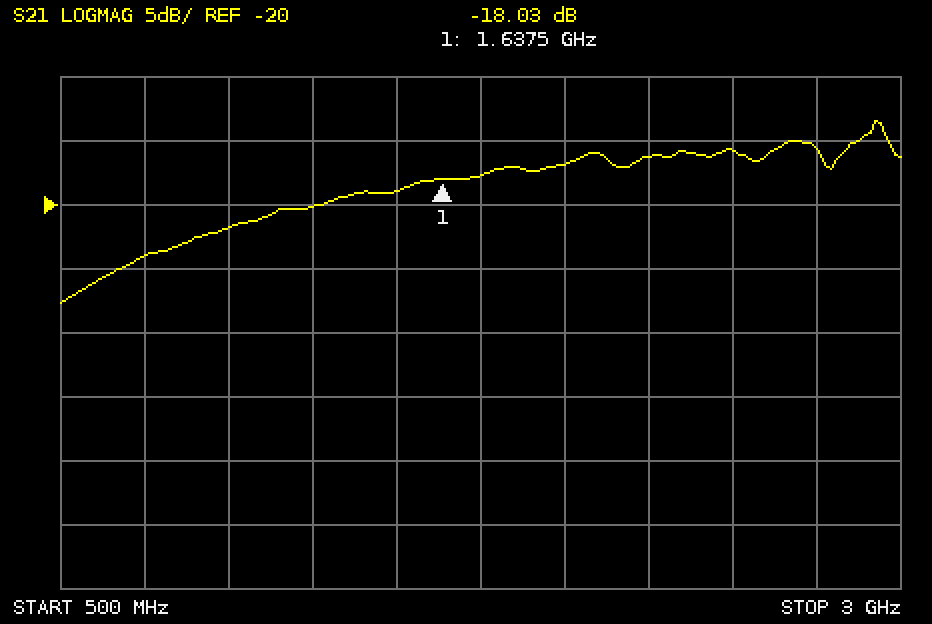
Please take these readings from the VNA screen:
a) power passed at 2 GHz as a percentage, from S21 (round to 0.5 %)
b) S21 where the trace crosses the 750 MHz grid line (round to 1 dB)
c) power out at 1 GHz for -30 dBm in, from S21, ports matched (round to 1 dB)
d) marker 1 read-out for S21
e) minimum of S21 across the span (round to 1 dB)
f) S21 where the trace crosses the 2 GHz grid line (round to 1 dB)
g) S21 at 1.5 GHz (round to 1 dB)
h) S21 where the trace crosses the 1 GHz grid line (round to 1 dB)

2.0 %
-24 dB
-52 dBm
-18.03 dB
-28 dB
-17 dB
-19 dB
-22 dB
